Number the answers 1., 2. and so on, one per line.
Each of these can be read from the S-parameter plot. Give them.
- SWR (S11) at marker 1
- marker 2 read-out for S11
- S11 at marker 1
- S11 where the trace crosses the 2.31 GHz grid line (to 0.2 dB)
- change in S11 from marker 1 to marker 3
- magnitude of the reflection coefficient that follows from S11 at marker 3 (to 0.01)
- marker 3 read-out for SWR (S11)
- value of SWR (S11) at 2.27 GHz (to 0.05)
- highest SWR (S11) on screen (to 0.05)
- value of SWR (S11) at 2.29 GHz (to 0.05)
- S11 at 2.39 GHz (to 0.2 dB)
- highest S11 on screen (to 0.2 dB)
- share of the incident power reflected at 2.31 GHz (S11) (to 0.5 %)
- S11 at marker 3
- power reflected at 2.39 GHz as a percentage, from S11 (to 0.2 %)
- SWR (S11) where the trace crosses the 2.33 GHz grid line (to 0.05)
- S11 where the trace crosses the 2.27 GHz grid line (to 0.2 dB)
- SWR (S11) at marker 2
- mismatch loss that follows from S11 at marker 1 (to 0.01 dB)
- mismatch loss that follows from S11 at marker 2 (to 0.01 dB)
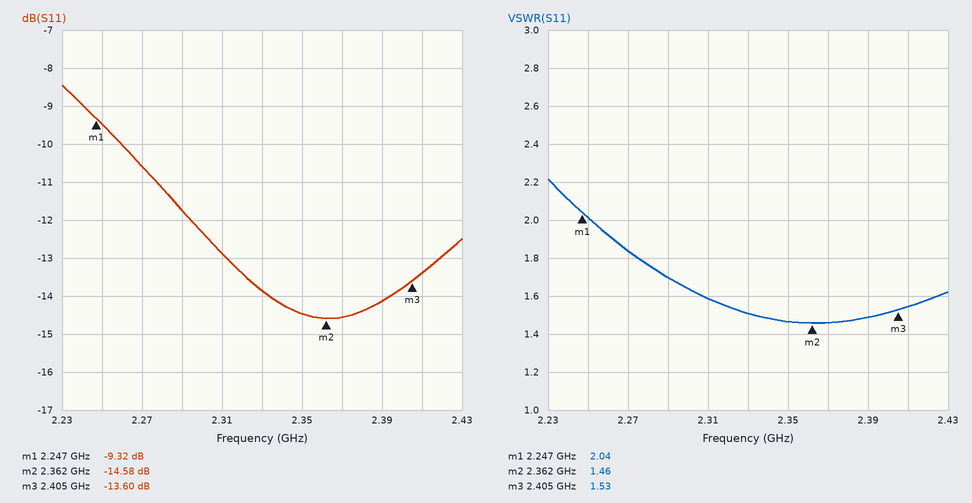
1. 2.04
2. -14.58 dB
3. -9.32 dB
4. -12.8 dB
5. -4.28 dB
6. 0.21
7. 1.53
8. 1.85
9. 2.20
10. 1.70
11. -14.2 dB
12. -8.4 dB
13. 5.0 %
14. -13.60 dB
15. 3.8 %
16. 1.50
17. -10.6 dB
18. 1.46
19. 0.54 dB
20. 0.15 dB
